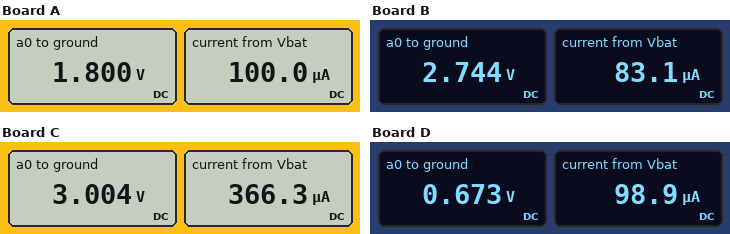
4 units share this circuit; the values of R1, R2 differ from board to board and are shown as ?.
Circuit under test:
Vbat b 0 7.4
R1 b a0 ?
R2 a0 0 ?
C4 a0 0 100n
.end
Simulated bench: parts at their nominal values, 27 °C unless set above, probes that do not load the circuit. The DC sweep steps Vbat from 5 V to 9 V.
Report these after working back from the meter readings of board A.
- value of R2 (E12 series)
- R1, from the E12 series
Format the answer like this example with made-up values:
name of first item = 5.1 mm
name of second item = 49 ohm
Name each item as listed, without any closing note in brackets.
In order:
value of R2 = 18 kΩ
R1, from the E12 series = 56 kΩ
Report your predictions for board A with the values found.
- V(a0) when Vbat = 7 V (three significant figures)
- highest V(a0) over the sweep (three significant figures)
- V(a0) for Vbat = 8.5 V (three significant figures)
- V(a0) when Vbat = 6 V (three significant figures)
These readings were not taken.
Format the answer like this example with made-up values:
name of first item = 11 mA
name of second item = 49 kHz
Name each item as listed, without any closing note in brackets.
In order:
V(a0) when Vbat = 7 V = 1.70 V
highest V(a0) over the sweep = 2.19 V
V(a0) for Vbat = 8.5 V = 2.07 V
V(a0) when Vbat = 6 V = 1.46 V
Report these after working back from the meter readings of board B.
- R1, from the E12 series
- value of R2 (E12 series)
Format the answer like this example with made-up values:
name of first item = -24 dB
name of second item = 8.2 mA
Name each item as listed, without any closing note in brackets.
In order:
R1, from the E12 series = 56 kΩ
value of R2 = 33 kΩ
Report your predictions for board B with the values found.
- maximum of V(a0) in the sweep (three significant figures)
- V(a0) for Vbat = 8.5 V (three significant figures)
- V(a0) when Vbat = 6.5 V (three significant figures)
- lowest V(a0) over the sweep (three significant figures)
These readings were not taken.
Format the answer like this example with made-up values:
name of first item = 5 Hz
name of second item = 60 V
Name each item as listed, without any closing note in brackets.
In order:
maximum of V(a0) in the sweep = 3.34 V
V(a0) for Vbat = 8.5 V = 3.15 V
V(a0) when Vbat = 6.5 V = 2.41 V
lowest V(a0) over the sweep = 1.85 V
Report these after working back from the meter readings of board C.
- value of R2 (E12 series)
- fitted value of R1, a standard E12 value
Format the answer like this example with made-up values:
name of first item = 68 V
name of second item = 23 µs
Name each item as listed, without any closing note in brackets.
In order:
value of R2 = 8.2 kΩ
fitted value of R1, a standard E12 value = 12 kΩ
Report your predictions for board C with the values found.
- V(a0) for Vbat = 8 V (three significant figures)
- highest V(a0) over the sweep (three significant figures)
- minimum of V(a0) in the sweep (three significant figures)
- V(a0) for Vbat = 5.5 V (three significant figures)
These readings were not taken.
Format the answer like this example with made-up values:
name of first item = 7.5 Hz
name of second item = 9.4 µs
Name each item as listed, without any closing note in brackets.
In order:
V(a0) for Vbat = 8 V = 3.25 V
highest V(a0) over the sweep = 3.65 V
minimum of V(a0) in the sweep = 2.03 V
V(a0) for Vbat = 5.5 V = 2.23 V
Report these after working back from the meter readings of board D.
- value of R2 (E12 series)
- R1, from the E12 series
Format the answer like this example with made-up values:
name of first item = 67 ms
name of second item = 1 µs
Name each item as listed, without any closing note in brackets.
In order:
value of R2 = 6.8 kΩ
R1, from the E12 series = 68 kΩ
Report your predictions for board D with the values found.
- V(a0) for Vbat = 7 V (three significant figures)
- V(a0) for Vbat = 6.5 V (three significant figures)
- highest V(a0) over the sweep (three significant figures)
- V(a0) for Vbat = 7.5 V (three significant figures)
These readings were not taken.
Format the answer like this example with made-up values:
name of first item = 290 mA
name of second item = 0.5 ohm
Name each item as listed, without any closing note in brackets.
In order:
V(a0) for Vbat = 7 V = 636 mV
V(a0) for Vbat = 6.5 V = 591 mV
highest V(a0) over the sweep = 818 mV
V(a0) for Vbat = 7.5 V = 682 mV
